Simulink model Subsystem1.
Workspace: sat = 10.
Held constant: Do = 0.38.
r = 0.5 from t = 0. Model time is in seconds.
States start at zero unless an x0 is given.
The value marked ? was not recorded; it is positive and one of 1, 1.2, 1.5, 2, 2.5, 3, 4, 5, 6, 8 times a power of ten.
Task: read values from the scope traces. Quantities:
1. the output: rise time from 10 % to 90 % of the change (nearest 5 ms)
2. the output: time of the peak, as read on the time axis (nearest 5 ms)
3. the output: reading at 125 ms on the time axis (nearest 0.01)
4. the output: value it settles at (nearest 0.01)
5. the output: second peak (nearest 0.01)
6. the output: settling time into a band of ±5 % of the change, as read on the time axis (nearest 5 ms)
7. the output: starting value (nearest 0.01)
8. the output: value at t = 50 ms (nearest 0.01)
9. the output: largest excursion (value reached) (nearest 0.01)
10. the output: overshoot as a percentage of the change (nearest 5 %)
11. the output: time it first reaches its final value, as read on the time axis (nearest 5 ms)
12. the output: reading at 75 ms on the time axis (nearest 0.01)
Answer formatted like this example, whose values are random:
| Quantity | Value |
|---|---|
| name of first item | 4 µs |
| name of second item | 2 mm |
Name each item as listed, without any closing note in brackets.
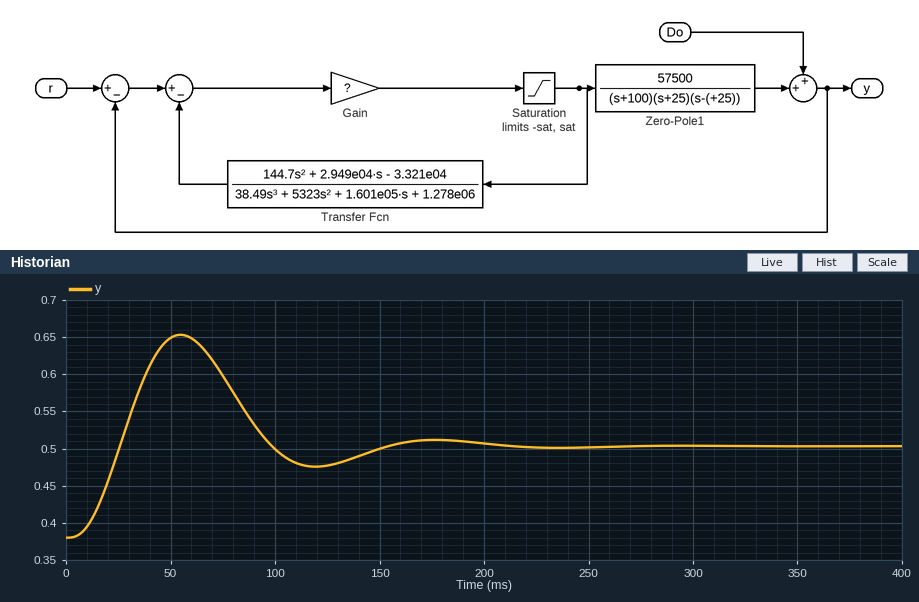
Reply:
| Quantity | Value |
|---|---|
| the output: rise time from 10 % to 90 % of the change | 15 ms |
| the output: time of the peak, as read on the time axis | 55 ms |
| the output: reading at 125 ms on the time axis | 0.48 |
| the output: value it settles at | 0.50 |
| the output: second peak | 0.51 |
| the output: settling time into a band of ±5 % of the change, as read on the time axis | 190 ms |
| the output: starting value | 0.38 |
| the output: value at t = 50 ms | 0.65 |
| the output: largest excursion (value reached) | 0.65 |
| the output: overshoot as a percentage of the change | 120 % |
| the output: time it first reaches its final value, as read on the time axis | 25 ms |
| the output: reading at 75 ms on the time axis | 0.60 |
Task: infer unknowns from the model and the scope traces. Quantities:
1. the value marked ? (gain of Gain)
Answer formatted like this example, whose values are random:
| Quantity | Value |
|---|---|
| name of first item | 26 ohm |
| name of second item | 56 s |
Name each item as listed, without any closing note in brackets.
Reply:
| Quantity | Value |
|---|---|
| the value marked ? | 20 |
